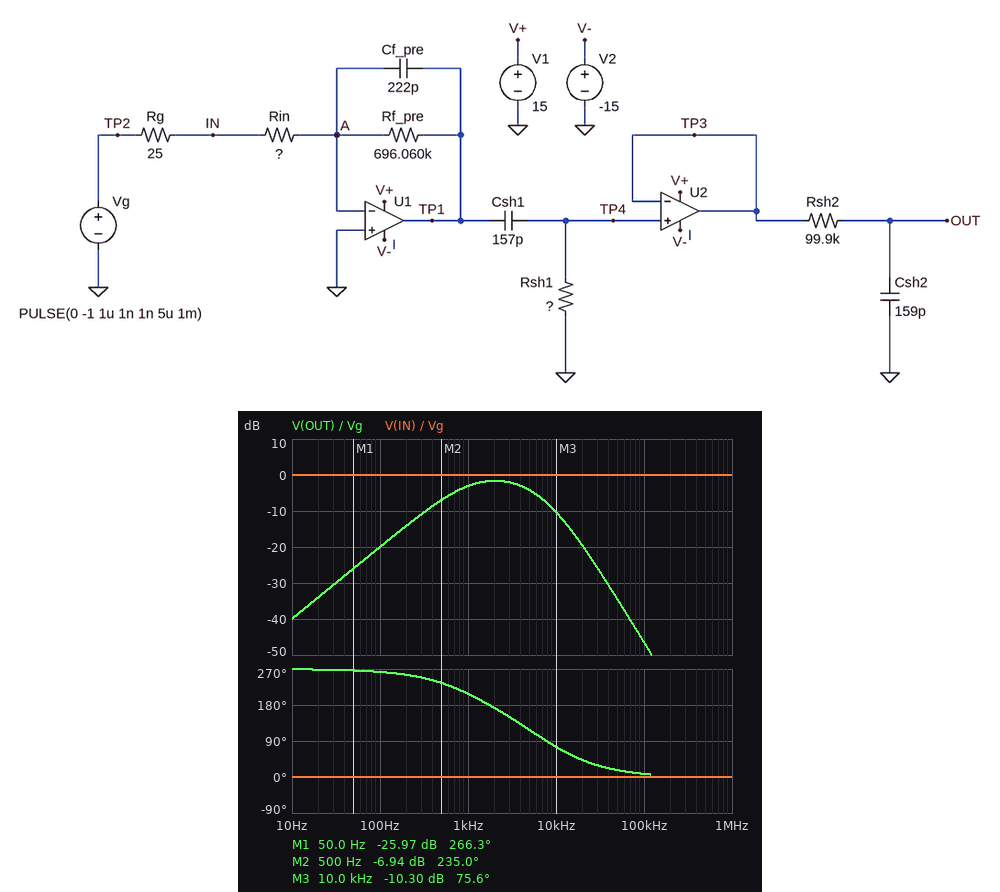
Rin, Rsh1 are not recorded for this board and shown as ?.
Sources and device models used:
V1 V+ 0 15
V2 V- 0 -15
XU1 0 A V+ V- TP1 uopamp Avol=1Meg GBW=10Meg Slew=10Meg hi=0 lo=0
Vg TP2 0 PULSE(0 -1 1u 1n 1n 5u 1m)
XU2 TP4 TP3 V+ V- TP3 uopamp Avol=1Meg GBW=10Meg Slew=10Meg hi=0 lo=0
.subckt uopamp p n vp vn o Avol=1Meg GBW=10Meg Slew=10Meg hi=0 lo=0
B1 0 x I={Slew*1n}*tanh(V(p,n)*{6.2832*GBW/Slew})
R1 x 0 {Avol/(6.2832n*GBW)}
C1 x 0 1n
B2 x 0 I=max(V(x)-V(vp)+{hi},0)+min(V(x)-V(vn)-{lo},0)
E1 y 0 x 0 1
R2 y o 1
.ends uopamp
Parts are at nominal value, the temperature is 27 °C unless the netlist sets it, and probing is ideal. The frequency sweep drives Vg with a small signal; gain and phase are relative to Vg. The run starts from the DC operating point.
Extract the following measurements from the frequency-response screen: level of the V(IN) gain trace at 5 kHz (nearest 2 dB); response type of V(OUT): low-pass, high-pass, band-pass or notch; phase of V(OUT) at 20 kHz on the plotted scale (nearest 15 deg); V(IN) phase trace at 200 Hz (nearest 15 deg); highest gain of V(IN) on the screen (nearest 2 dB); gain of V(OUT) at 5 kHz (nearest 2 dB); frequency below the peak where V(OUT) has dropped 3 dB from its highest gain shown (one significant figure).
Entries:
0 dB
band-pass
45 deg
0 deg
0 dB
-4 dB
700 Hz
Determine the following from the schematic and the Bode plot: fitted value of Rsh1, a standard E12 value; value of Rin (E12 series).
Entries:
220 kΩ
150 kΩ
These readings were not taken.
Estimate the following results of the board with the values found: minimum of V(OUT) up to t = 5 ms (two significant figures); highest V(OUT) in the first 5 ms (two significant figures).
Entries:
-14 mV
70 mV
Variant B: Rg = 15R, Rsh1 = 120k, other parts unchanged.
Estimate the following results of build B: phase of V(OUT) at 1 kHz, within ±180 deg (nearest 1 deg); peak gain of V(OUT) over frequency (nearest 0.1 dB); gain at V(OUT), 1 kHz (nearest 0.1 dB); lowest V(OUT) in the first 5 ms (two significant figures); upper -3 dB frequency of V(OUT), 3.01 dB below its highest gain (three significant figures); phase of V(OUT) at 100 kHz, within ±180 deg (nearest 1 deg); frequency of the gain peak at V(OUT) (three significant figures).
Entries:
-147 deg
-6.3 dB
-8.2 dB
-9.4 mV
7.26 kHz
10 deg
2.53 kHz
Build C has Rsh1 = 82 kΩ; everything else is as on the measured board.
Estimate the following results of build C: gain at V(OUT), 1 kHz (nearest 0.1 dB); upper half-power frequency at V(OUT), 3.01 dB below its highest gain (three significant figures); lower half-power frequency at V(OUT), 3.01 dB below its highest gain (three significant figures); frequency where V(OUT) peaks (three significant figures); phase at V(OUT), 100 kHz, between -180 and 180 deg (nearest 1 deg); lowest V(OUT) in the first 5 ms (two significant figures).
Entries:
-11.5 dB
8.51 kHz
828 Hz
2.79 kHz
12 deg
-7.0 mV
